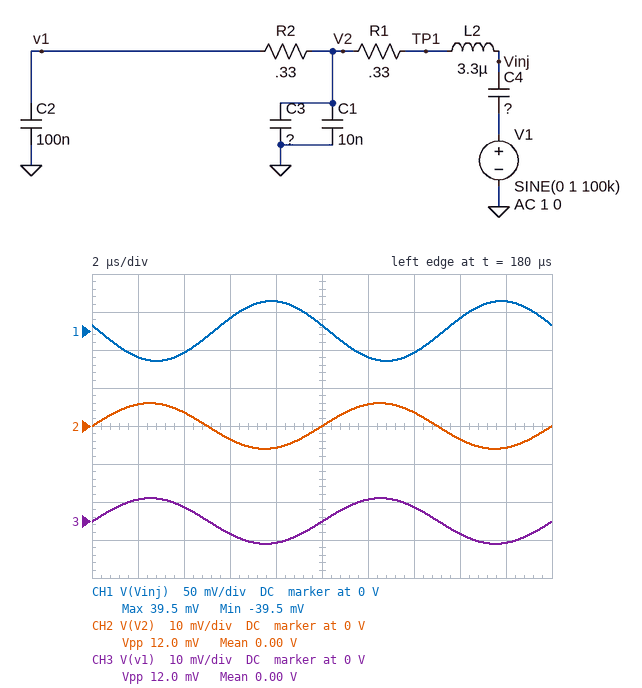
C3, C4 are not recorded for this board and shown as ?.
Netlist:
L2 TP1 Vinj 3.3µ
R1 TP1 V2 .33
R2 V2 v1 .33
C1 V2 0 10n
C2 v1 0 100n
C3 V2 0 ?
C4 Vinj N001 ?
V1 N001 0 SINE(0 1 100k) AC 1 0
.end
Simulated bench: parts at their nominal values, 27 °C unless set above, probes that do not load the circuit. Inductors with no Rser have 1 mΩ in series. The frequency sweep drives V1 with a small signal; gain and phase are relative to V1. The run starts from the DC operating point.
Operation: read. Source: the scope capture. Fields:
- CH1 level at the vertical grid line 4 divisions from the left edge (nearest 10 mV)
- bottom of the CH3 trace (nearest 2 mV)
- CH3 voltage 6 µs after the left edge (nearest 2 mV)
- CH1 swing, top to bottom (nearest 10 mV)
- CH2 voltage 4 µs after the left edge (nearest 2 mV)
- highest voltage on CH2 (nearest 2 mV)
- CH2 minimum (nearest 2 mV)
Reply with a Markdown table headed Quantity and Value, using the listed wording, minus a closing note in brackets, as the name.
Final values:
| Quantity | Value |
|---|---|
| CH1 level at the vertical grid line 4 divisions from the left edge | 40 mV |
| bottom of the CH3 trace | -6 mV |
| CH3 voltage 6 µs after the left edge | -4 mV |
| CH1 swing, top to bottom | 80 mV |
| CH2 voltage 4 µs after the left edge | 4 mV |
| highest voltage on CH2 | 6 mV |
| CH2 minimum | -6 mV |
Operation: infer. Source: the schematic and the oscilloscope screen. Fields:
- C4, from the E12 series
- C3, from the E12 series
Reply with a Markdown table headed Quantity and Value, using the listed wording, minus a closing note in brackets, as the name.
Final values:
| Quantity | Value |
|---|---|
| C4, from the E12 series | 33 nF |
| C3, from the E12 series | 5.6 µF |
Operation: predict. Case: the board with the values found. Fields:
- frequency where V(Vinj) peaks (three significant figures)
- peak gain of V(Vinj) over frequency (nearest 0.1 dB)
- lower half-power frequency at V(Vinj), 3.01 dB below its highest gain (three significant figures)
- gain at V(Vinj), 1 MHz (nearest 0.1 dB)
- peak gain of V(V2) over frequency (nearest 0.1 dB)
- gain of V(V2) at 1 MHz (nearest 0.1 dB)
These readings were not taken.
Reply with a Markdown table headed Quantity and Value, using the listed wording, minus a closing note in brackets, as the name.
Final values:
| Quantity | Value |
|---|---|
| frequency where V(Vinj) peaks | 484 kHz |
| peak gain of V(Vinj) over frequency | 29.6 dB |
| lower half-power frequency at V(Vinj), 3.01 dB below its highest gain | 476 kHz |
| gain at V(Vinj), 1 MHz | 2.3 dB |
| peak gain of V(V2) over frequency | -15.2 dB |
| gain of V(V2) at 1 MHz | -55.1 dB |
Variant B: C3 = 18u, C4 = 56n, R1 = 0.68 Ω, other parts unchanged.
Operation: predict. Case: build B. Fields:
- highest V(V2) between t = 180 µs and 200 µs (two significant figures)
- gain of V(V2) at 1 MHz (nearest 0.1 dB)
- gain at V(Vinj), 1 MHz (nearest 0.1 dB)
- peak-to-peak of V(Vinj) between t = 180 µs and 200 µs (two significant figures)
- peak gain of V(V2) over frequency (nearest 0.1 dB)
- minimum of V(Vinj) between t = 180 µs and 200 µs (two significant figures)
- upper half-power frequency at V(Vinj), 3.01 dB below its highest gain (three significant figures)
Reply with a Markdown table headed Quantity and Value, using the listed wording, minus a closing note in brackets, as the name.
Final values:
| Quantity | Value |
|---|---|
| highest V(V2) between t = 180 µs and 200 µs | 3.3 mV |
| gain of V(V2) at 1 MHz | -66.2 dB |
| gain at V(Vinj), 1 MHz | 1.3 dB |
| peak-to-peak of V(Vinj) between t = 180 µs and 200 µs | 160 mV |
| peak gain of V(V2) over frequency | -29.2 dB |
| minimum of V(Vinj) between t = 180 µs and 200 µs | -79 mV |
| upper half-power frequency at V(Vinj), 3.01 dB below its highest gain | 389 kHz |
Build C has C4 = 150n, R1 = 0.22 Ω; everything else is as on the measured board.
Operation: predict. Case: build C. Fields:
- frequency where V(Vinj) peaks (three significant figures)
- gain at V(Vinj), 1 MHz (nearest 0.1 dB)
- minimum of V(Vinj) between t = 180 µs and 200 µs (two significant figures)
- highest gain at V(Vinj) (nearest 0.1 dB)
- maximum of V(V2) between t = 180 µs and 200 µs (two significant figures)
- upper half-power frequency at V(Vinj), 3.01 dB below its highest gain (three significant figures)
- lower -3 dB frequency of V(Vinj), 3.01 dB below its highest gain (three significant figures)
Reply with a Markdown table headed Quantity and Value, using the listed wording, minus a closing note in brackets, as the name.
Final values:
| Quantity | Value |
|---|---|
| frequency where V(Vinj) peaks | 229 kHz |
| gain at V(Vinj), 1 MHz | 0.5 dB |
| minimum of V(Vinj) between t = 180 µs and 200 µs | -210 mV |
| highest gain at V(Vinj) | 26.4 dB |
| maximum of V(V2) between t = 180 µs and 200 µs | 32 mV |
| upper half-power frequency at V(Vinj), 3.01 dB below its highest gain | 235 kHz |
| lower -3 dB frequency of V(Vinj), 3.01 dB below its highest gain | 224 kHz |
